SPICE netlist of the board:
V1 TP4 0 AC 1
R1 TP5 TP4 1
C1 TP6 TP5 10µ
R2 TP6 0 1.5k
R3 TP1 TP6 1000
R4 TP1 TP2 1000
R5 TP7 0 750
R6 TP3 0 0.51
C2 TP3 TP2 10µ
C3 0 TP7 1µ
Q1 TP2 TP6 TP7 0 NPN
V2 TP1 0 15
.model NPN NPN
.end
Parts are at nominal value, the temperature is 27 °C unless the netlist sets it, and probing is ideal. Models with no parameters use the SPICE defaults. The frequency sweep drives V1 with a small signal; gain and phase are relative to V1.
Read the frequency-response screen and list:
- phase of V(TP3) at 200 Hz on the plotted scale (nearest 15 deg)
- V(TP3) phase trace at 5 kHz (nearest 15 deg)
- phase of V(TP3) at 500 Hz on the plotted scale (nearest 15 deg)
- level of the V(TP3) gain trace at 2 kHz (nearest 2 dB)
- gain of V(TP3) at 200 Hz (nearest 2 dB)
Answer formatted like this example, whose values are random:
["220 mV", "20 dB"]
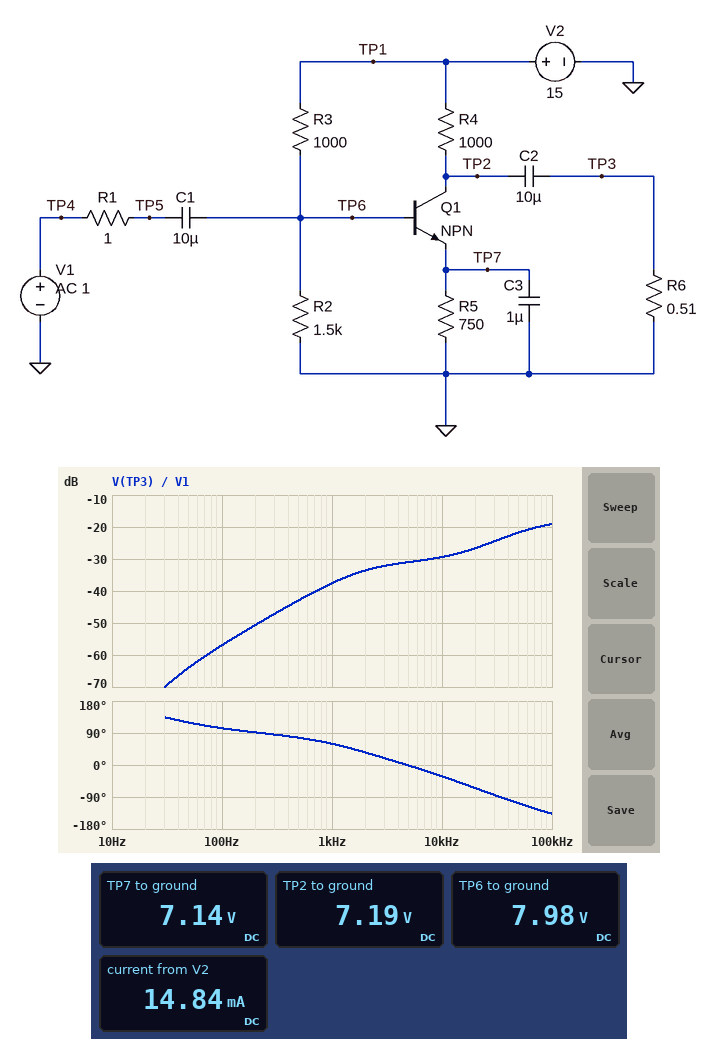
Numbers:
["90 deg", "0 deg", "75 deg", "-34 dB", "-50 dB"]
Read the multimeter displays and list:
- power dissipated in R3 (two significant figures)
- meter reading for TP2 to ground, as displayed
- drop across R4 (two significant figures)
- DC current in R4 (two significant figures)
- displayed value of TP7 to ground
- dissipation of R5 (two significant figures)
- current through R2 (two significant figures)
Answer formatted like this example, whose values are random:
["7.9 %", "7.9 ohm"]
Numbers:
["49 mW", "7.19 V", "7.8 V", "7.8 mA", "7.14 V", "68 mW", "5.3 mA"]
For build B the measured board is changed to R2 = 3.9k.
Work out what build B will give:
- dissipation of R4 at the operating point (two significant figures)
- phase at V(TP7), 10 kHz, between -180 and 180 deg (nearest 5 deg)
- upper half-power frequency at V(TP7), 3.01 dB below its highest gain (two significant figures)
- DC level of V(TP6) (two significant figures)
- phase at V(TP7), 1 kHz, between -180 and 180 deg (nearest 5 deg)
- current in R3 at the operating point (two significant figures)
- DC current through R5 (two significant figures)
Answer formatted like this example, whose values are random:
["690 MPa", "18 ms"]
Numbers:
["48 mW", "0 deg", "89 kHz", "8.9 V", "5 deg", "6.1 mA", "11 mA"]
